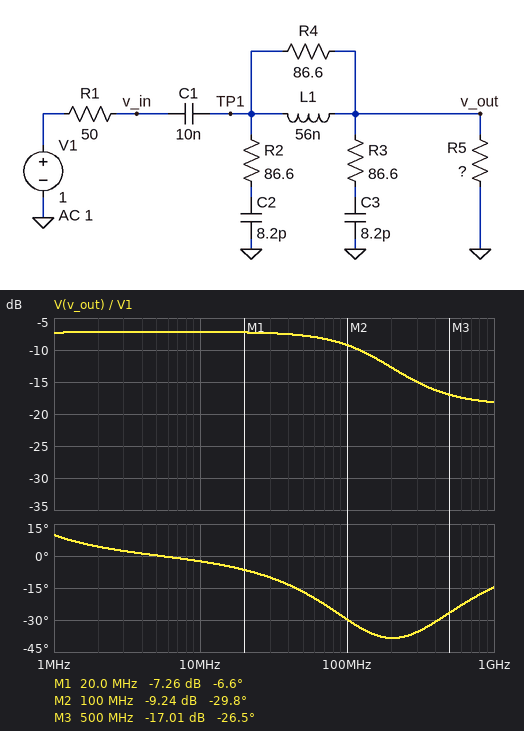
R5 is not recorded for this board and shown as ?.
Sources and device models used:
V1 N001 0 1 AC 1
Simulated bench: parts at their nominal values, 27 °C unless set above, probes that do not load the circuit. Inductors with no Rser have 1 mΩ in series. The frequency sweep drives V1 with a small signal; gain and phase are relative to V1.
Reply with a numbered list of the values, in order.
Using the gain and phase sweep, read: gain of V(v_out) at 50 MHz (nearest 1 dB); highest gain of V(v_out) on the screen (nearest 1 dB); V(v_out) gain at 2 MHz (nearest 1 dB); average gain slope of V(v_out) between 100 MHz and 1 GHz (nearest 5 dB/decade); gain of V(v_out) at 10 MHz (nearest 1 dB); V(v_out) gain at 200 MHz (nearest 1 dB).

1. -8 dB
2. -7 dB
3. -7 dB
4. -10 dB/decade
5. -7 dB
6. -13 dB
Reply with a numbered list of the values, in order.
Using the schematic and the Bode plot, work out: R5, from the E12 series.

1. 39 Ω
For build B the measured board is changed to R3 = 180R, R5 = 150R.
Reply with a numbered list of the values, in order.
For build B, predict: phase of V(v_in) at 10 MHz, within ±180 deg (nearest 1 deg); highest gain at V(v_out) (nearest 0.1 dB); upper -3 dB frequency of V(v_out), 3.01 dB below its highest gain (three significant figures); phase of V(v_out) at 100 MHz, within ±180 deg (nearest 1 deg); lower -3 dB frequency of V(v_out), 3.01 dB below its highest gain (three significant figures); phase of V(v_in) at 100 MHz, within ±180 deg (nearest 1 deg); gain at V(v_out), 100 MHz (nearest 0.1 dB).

1. -2 deg
2. -2.5 dB
3. 134 MHz
4. -25 deg
5. 79.4 kHz
6. -8 deg
7. -4.5 dB
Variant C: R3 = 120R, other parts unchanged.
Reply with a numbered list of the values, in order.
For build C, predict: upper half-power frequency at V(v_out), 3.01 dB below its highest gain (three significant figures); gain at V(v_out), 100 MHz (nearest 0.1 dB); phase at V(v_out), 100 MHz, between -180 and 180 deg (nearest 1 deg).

1. 124 MHz
2. -9.3 dB
3. -29 deg
